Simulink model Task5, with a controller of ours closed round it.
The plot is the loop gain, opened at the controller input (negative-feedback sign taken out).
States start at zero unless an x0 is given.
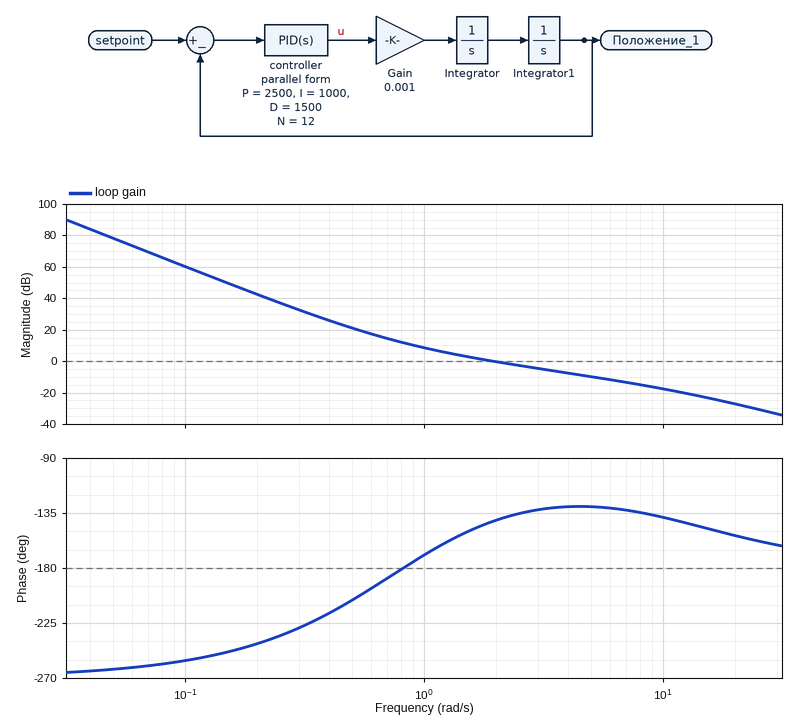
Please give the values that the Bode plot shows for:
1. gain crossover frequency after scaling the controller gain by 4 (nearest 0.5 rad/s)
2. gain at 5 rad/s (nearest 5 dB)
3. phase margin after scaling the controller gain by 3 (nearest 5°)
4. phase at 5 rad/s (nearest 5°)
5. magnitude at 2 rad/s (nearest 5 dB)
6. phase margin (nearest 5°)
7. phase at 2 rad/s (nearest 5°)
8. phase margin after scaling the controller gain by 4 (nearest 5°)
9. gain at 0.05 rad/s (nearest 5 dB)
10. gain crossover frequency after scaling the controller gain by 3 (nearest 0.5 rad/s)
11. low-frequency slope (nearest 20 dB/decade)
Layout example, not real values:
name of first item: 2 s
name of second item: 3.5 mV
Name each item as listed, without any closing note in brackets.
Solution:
gain crossover frequency after scaling the controller gain by 4: 6.0 rad/s
gain at 5 rad/s: -10 dB
phase margin after scaling the controller gain by 3: 50°
phase at 5 rad/s: -130°
magnitude at 2 rad/s: 0 dB
phase margin: 40°
phase at 2 rad/s: -140°
phase margin after scaling the controller gain by 4: 50°
gain at 0.05 rad/s: 80 dB
gain crossover frequency after scaling the controller gain by 3: 5.0 rad/s
low-frequency slope: -60 dB/decade
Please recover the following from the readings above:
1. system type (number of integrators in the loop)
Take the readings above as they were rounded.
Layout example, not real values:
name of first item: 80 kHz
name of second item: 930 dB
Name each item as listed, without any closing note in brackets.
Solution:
system type: 3
